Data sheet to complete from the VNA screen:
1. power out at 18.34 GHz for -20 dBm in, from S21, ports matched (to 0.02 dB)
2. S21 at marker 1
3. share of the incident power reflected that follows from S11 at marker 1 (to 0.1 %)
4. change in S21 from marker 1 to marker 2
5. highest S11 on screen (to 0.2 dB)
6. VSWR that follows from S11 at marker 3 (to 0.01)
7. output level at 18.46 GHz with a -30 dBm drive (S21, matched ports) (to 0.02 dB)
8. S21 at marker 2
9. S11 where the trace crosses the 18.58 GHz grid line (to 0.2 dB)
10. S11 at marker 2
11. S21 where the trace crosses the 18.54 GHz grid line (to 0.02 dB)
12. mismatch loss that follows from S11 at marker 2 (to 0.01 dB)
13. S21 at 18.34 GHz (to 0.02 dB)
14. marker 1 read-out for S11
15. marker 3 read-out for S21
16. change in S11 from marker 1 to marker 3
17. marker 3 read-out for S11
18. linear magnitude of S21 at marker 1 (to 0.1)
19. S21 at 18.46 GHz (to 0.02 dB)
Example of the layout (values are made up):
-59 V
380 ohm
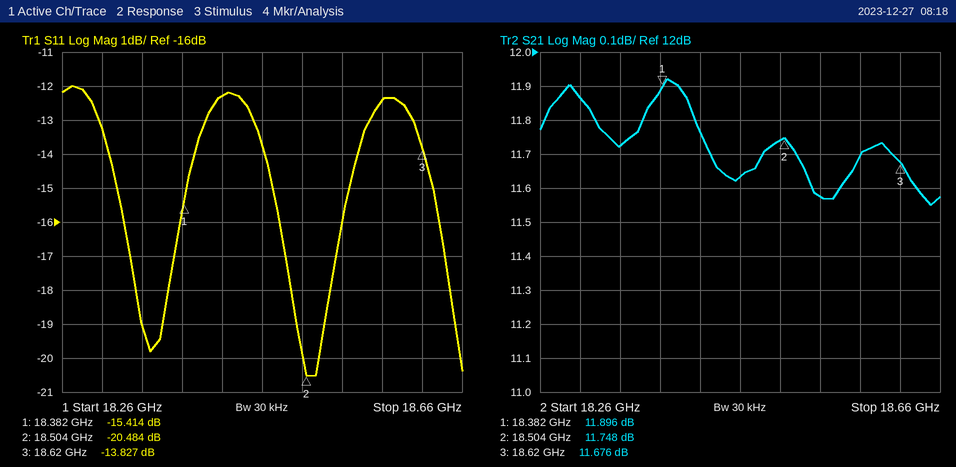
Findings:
-8.28 dBm
11.896 dB
2.9 %
-0.148 dB
-12.0 dB
1.51
-18.36 dBm
11.748 dB
-12.4 dB
-20.484 dB
11.58 dB
0.04 dB
11.72 dB
-15.414 dB
11.676 dB
1.587 dB
-13.827 dB
3.9
11.64 dB
